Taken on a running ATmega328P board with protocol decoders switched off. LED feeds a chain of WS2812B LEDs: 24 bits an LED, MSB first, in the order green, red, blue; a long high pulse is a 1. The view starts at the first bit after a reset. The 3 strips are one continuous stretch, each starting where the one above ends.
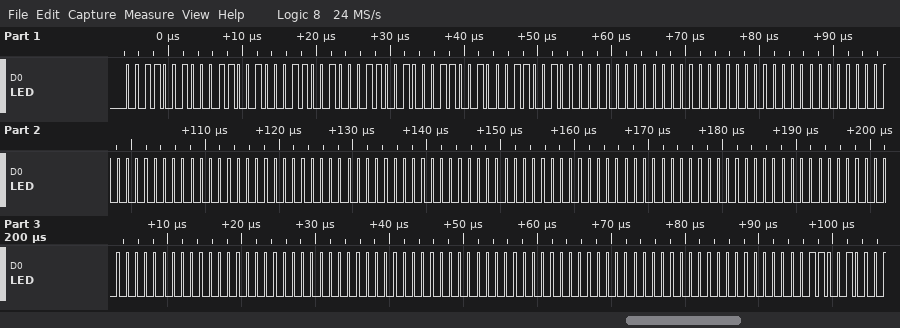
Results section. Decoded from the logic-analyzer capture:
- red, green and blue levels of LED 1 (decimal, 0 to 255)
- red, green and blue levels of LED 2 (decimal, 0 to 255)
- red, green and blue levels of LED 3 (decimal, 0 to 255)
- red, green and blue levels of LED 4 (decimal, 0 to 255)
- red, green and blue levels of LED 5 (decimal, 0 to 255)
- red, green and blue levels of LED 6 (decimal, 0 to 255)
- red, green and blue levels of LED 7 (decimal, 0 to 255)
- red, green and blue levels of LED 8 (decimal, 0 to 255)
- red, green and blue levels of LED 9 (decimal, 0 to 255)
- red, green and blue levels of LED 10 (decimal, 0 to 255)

50, 50, 50
50, 50, 50
0, 0, 0
0, 0, 0
0, 0, 0
0, 0, 0
0, 0, 0
0, 0, 0
0, 0, 0
0, 0, 0
